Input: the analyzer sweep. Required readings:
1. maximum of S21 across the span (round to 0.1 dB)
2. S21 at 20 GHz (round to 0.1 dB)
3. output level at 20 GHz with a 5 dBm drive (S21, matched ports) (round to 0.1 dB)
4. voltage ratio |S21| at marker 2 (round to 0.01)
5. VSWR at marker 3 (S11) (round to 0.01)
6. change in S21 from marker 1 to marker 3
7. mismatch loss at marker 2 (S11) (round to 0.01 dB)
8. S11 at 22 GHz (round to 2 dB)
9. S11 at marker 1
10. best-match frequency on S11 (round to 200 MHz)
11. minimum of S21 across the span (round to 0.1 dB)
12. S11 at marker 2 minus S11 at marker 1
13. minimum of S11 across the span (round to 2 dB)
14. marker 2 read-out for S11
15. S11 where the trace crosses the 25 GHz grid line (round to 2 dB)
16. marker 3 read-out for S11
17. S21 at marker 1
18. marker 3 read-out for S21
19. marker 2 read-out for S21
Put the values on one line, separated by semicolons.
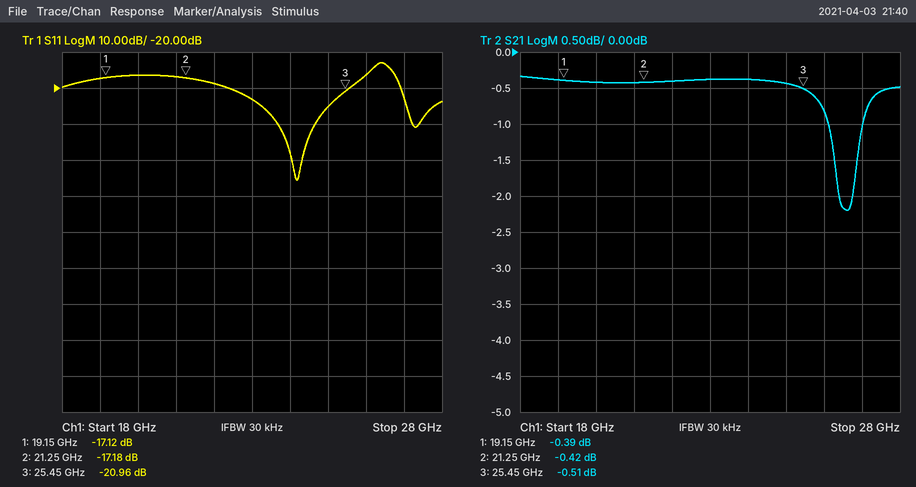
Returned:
-0.3 dB; -0.4 dB; 4.6 dBm; 0.95; 1.20; -0.12 dB; 0.08 dB; -18 dB; -17.12 dB; 24.2 GHz; -2.2 dB; -0.06 dB; -46 dB; -17.18 dB; -26 dB; -20.96 dB; -0.39 dB; -0.51 dB; -0.42 dB
